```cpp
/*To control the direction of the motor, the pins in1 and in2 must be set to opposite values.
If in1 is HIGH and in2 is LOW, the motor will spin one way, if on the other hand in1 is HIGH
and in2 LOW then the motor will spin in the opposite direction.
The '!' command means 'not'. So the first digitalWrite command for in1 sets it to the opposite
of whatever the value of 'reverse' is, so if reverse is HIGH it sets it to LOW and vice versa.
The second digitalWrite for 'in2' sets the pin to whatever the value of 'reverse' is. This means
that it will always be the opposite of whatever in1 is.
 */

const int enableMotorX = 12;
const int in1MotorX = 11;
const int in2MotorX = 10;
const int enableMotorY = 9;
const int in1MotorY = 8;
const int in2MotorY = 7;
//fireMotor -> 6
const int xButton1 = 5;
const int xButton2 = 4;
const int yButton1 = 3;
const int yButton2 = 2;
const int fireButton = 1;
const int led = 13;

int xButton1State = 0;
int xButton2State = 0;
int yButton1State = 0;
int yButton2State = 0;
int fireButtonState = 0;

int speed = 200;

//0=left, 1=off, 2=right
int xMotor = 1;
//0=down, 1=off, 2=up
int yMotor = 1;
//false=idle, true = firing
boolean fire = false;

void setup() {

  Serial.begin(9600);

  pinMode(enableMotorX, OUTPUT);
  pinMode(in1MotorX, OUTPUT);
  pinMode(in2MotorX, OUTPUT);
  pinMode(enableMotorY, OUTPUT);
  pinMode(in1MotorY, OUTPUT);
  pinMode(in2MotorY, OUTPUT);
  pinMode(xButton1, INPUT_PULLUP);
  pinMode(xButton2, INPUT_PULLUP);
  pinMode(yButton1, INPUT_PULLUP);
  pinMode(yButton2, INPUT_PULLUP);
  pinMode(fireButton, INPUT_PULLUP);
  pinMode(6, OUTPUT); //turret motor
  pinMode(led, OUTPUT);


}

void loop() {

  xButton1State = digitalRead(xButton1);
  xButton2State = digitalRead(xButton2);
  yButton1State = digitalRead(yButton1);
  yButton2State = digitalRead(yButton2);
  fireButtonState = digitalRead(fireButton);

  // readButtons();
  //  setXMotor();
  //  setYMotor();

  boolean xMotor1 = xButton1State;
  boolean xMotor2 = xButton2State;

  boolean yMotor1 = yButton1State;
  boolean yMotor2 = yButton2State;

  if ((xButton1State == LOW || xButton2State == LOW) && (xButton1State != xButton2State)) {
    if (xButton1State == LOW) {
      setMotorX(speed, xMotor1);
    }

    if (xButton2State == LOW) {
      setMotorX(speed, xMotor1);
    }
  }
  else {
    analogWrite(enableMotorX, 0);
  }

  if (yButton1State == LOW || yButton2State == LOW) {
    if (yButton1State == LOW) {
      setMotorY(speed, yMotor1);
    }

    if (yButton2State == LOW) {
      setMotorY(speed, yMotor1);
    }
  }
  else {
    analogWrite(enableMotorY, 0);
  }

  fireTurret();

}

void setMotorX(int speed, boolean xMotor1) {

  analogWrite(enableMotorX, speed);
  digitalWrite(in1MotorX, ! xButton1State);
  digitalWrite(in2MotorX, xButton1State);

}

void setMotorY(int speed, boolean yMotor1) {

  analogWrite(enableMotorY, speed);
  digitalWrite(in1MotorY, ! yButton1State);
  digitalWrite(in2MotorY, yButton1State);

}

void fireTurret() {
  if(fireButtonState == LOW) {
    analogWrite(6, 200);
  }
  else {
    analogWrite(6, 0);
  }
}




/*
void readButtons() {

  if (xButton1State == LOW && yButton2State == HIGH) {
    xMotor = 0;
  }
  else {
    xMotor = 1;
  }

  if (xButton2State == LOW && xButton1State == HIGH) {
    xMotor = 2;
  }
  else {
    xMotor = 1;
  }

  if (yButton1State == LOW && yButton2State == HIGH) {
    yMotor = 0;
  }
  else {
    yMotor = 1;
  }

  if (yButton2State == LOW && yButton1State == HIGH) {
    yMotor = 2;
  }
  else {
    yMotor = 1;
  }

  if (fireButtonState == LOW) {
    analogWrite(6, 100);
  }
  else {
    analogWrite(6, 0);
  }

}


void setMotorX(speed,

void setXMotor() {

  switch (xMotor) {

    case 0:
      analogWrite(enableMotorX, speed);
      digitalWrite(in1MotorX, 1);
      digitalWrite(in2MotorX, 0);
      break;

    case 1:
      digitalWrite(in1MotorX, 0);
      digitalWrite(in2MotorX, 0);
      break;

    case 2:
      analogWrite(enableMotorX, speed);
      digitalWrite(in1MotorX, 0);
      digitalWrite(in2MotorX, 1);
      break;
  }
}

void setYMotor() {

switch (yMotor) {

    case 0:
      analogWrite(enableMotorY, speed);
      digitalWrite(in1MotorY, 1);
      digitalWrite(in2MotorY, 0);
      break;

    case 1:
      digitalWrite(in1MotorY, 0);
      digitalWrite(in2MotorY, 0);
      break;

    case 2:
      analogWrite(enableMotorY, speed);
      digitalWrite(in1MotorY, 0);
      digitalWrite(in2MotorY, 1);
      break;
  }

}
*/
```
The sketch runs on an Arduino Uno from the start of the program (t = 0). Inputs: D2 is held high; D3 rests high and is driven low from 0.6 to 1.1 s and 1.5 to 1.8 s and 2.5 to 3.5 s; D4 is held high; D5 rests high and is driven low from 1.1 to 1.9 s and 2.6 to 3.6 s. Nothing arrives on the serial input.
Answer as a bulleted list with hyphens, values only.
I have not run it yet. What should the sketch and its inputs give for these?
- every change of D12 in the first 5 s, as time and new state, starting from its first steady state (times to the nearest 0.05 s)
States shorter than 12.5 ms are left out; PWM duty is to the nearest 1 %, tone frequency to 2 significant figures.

- 0 s low; 1.1 s high; 1.9 s low; 2.6 s high; 3.6 s low
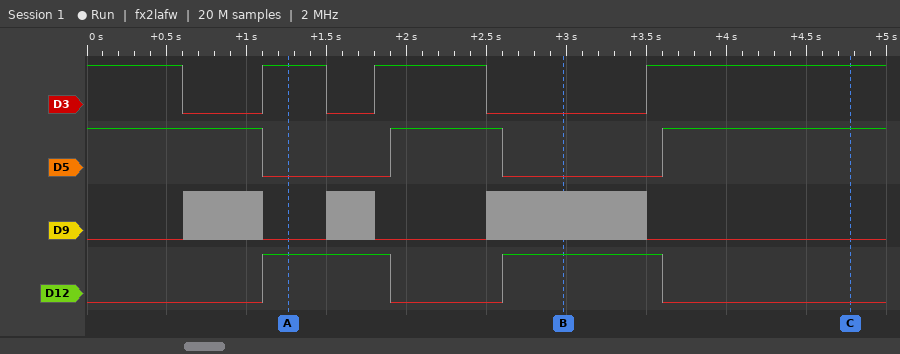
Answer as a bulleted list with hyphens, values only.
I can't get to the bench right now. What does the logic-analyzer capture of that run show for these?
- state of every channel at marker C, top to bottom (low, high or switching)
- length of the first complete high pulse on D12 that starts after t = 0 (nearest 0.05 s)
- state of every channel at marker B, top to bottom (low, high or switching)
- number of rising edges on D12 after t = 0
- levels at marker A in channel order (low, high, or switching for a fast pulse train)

- D3 high, D5 high, D9 low, D12 low
- 0.80 s
- D3 low, D5 low, D9 switching, D12 high
- 2
- D3 high, D5 low, D9 low, D12 high
